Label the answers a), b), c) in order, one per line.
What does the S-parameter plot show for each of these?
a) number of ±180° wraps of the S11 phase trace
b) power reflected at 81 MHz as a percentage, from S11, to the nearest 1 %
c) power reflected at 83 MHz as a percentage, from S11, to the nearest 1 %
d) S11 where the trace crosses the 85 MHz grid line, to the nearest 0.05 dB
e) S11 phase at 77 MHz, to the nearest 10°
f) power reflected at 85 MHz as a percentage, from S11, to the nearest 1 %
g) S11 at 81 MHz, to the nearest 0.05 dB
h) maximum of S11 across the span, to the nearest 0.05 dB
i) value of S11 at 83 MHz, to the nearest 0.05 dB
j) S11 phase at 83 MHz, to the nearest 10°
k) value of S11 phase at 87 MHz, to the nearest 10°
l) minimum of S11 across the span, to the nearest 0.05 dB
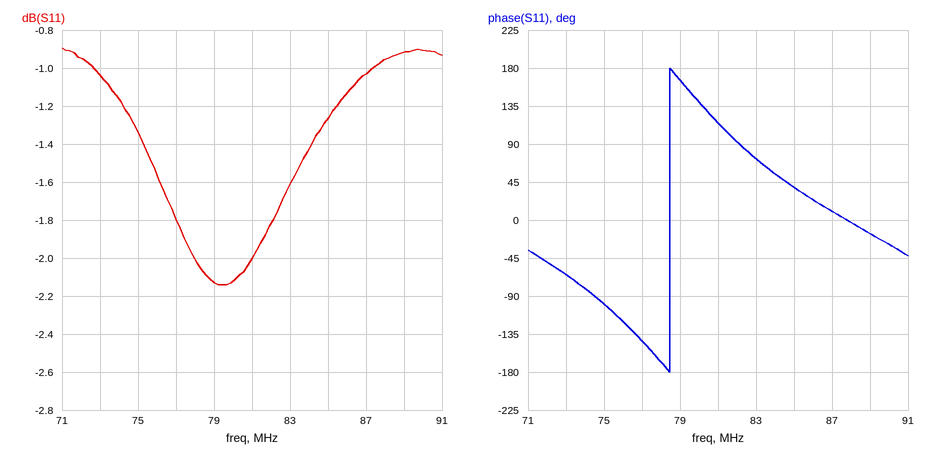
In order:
a) 1
b) 63 %
c) 69 %
d) -1.25 dB
e) -140°
f) 75 %
g) -2.00 dB
h) -0.90 dB
i) -1.60 dB
j) 70°
k) 10°
l) -2.15 dB
